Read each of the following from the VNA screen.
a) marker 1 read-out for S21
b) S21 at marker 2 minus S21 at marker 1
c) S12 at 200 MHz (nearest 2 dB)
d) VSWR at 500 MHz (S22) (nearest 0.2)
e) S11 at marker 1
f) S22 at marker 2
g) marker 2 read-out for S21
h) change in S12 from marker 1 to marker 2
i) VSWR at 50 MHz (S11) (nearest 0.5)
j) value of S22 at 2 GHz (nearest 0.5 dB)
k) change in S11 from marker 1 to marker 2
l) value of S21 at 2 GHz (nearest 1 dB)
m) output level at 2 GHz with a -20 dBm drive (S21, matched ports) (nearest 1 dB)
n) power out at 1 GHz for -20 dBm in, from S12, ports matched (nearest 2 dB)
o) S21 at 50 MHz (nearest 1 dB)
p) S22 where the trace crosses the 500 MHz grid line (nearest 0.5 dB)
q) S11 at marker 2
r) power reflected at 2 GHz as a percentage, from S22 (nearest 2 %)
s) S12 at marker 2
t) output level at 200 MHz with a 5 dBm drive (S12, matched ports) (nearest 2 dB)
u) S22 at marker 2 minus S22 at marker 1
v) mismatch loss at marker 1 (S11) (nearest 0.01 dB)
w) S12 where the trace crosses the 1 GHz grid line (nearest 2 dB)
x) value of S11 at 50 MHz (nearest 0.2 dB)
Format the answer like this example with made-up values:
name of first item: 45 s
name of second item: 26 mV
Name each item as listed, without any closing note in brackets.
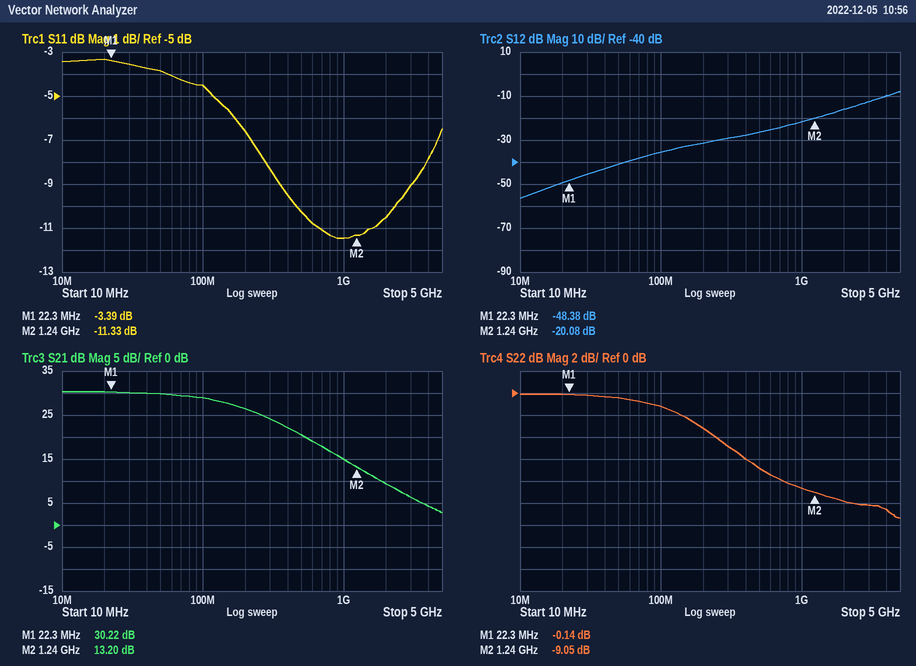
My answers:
marker 1 read-out for S21: 30.22 dB
S21 at marker 2 minus S21 at marker 1: -17.02 dB
S12 at 200 MHz: -32 dB
VSWR at 500 MHz (S22): 2.6
S11 at marker 1: -3.39 dB
S22 at marker 2: -9.05 dB
marker 2 read-out for S21: 13.20 dB
change in S12 from marker 1 to marker 2: 28.30 dB
VSWR at 50 MHz (S11): 4.5
value of S22 at 2 GHz: -10.0 dB
change in S11 from marker 1 to marker 2: -7.94 dB
value of S21 at 2 GHz: 9 dB
output level at 2 GHz with a -20 dBm drive (S21, matched ports): -11 dBm
power out at 1 GHz for -20 dBm in, from S12, ports matched: -42 dBm
S21 at 50 MHz: 30 dB
S22 where the trace crosses the 500 MHz grid line: -7.0 dB
S11 at marker 2: -11.33 dB
power reflected at 2 GHz as a percentage, from S22: 10 %
S12 at marker 2: -20.08 dB
output level at 200 MHz with a 5 dBm drive (S12, matched ports): -26 dBm
S22 at marker 2 minus S22 at marker 1: -8.91 dB
mismatch loss at marker 1 (S11): 2.66 dB
S12 where the trace crosses the 1 GHz grid line: -22 dB
value of S11 at 50 MHz: -3.8 dB
